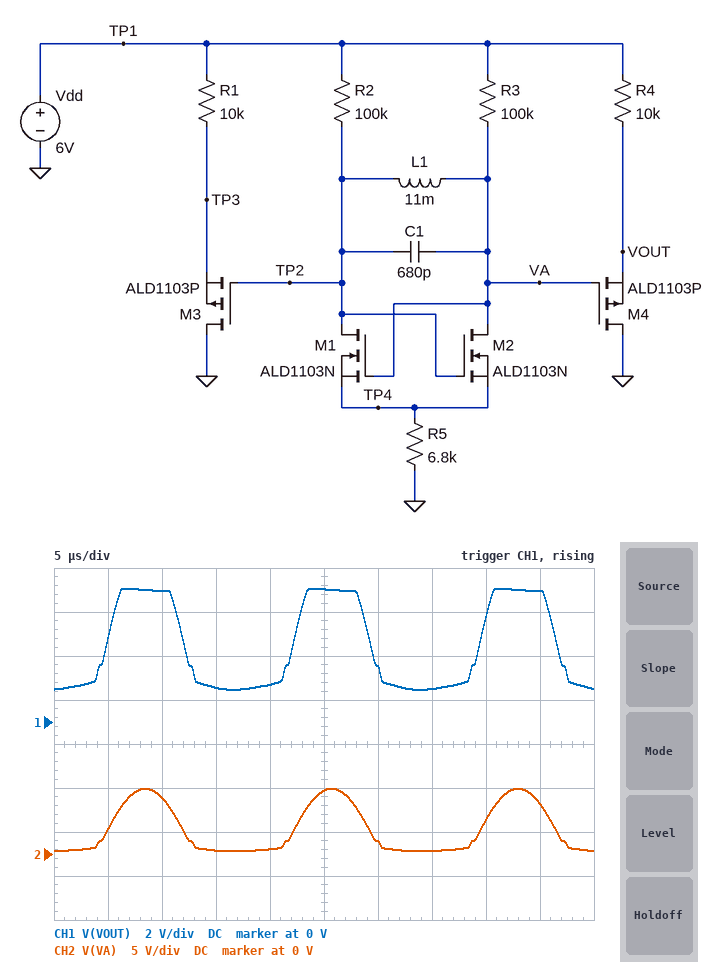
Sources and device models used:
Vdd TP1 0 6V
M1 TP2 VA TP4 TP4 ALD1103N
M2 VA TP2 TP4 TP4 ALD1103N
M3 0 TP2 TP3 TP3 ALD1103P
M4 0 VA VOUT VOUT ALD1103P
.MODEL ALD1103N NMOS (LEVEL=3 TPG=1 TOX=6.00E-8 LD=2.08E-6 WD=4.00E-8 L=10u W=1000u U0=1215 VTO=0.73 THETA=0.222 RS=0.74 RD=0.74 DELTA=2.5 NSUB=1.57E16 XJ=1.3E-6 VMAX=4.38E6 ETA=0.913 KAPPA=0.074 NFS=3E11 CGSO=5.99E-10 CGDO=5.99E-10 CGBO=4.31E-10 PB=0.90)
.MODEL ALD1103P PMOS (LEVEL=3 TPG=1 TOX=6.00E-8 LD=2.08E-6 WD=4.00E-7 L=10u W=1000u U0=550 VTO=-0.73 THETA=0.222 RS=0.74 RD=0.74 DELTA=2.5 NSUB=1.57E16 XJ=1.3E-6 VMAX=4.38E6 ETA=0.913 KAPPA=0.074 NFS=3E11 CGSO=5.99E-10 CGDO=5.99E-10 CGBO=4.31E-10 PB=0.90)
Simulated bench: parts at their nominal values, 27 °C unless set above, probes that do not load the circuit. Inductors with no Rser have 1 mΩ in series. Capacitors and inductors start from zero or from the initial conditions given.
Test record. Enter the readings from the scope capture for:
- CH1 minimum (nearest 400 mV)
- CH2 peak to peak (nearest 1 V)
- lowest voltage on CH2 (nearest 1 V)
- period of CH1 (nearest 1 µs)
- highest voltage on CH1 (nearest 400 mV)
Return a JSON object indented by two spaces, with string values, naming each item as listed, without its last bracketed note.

{
  "CH1 minimum": "1.6 V",
  "CH2 peak to peak": "7 V",
  "lowest voltage on CH2": "0 V",
  "period of CH1": "17 µs",
  "highest voltage on CH1": "6.0 V"
}
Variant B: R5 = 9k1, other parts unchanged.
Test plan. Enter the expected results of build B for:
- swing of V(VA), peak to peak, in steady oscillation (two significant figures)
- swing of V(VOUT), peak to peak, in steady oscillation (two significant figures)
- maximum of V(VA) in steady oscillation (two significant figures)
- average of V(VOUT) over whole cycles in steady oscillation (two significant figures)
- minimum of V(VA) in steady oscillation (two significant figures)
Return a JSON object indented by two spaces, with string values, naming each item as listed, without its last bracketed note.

{
  "swing of V(VA), peak to peak, in steady oscillation": "7.0 V",
  "swing of V(VOUT), peak to peak, in steady oscillation": "4.5 V",
  "maximum of V(VA) in steady oscillation": "7.4 V",
  "average of V(VOUT) over whole cycles in steady oscillation": "3.5 V",
  "minimum of V(VA) in steady oscillation": "380 mV"
}
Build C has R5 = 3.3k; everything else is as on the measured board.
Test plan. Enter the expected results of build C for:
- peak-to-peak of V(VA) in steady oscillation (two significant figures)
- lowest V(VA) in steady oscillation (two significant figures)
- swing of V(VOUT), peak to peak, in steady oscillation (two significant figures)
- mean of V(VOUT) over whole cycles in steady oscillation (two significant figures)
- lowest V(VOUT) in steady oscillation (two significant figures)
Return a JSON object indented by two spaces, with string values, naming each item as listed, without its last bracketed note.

{
  "peak-to-peak of V(VA) in steady oscillation": "7.4 V",
  "lowest V(VA) in steady oscillation": "140 mV",
  "swing of V(VOUT), peak to peak, in steady oscillation": "4.7 V",
  "mean of V(VOUT) over whole cycles in steady oscillation": "3.2 V",
  "lowest V(VOUT) in steady oscillation": "1.3 V"
}
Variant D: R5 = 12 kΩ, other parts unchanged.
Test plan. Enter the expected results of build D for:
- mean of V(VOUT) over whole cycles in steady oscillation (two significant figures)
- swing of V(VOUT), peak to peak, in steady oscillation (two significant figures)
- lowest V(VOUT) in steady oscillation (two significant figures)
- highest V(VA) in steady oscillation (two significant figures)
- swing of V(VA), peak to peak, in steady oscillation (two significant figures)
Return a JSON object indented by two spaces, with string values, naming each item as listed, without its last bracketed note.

{
  "mean of V(VOUT) over whole cycles in steady oscillation": "3.6 V",
  "swing of V(VOUT), peak to peak, in steady oscillation": "4.4 V",
  "lowest V(VOUT) in steady oscillation": "1.7 V",
  "highest V(VA) in steady oscillation": "7.3 V",
  "swing of V(VA), peak to peak, in steady oscillation": "6.8 V"
}
